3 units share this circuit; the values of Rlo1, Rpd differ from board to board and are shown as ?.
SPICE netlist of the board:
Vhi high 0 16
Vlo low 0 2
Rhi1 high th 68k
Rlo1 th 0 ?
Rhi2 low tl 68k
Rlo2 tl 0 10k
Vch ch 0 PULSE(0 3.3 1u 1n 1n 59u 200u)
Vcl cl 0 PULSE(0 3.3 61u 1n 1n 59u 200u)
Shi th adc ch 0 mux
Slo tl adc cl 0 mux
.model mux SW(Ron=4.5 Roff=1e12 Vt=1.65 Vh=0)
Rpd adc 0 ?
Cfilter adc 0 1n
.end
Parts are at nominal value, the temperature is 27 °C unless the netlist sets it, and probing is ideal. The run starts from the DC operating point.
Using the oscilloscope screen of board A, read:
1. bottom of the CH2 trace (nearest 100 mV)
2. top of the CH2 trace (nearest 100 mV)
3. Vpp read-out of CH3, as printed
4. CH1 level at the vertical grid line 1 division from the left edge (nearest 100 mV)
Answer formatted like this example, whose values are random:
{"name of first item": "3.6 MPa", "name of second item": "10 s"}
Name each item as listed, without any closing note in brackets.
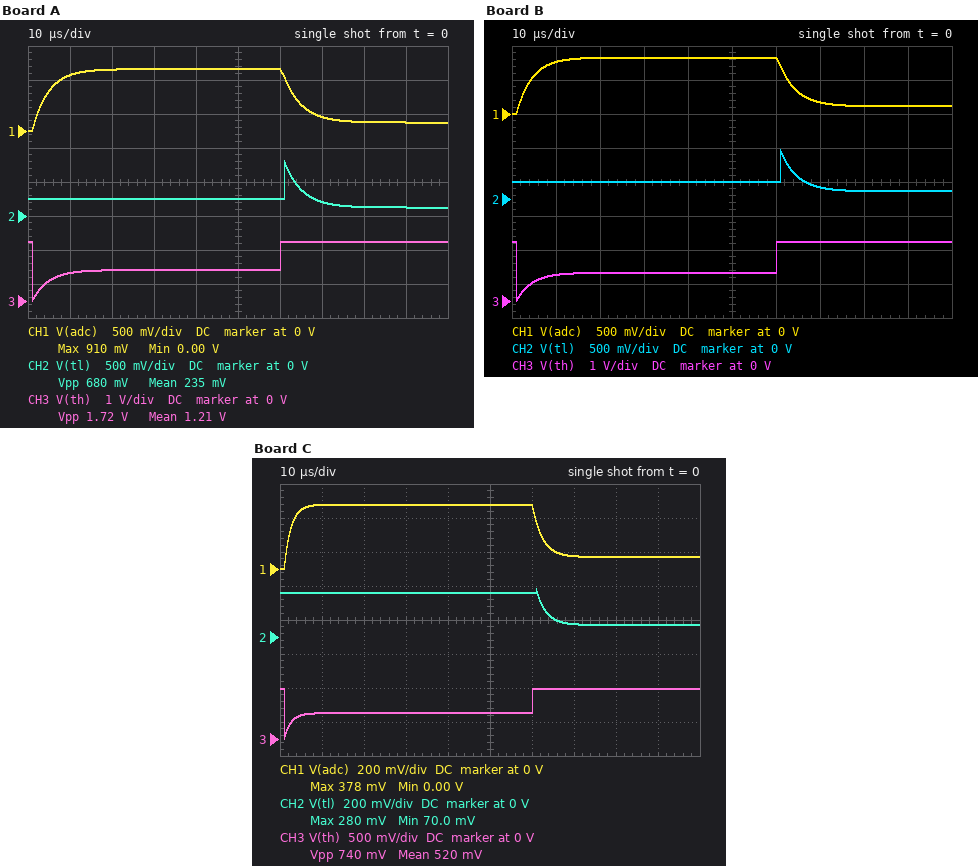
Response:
{"bottom of the CH2 trace": "100 mV", "top of the CH2 trace": "800 mV", "Vpp read-out of CH3, as printed": "1.72 V", "CH1 level at the vertical grid line 1 division from the left edge": "800 mV"}
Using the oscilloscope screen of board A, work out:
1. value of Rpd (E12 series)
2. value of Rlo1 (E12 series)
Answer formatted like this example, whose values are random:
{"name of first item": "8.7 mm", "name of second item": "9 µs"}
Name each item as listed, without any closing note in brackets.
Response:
{"value of Rpd": "8.2 kΩ", "value of Rlo1": "8.2 kΩ"}
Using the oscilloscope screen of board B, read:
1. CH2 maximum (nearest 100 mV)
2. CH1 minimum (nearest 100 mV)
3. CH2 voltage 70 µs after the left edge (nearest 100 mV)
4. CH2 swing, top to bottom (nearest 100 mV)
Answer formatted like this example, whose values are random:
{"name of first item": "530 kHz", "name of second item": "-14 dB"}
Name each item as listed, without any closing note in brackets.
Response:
{"CH2 maximum": "700 mV", "CH1 minimum": "0 V", "CH2 voltage 70 µs after the left edge": "200 mV", "CH2 swing, top to bottom": "600 mV"}
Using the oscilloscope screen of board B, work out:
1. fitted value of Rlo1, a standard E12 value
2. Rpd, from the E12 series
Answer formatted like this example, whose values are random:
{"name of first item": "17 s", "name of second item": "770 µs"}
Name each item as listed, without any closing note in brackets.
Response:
{"fitted value of Rlo1, a standard E12 value": "8.2 kΩ", "Rpd, from the E12 series": "6.8 kΩ"}
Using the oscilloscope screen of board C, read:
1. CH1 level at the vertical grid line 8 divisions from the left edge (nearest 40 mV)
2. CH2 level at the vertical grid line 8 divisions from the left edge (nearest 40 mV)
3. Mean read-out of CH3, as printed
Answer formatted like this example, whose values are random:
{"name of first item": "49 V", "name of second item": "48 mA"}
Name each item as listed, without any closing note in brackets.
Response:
{"CH1 level at the vertical grid line 8 divisions from the left edge": "80 mV", "CH2 level at the vertical grid line 8 divisions from the left edge": "80 mV", "Mean read-out of CH3, as printed": "520 mV"}
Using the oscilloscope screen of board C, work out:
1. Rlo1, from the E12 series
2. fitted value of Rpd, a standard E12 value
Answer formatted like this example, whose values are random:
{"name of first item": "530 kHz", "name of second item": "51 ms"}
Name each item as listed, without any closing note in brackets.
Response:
{"Rlo1, from the E12 series": "3.3 kΩ", "fitted value of Rpd, a standard E12 value": "3.3 kΩ"}
